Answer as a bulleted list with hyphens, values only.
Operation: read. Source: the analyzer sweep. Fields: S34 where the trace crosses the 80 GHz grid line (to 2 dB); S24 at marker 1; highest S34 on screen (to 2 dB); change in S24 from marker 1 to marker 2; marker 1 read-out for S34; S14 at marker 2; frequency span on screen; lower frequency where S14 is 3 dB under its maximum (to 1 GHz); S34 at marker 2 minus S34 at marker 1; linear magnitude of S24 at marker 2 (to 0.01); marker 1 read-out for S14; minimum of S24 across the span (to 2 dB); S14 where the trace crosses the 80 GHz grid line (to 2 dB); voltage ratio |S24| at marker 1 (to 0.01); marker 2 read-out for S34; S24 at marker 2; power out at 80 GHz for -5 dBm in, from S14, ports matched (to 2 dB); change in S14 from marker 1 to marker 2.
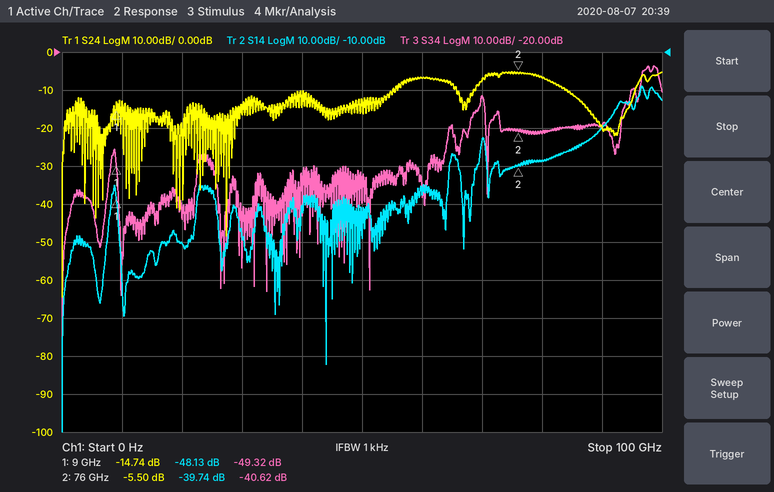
- -42 dB
- -14.74 dB
- -24 dB
- 9.24 dB
- -49.32 dB
- -39.74 dB
- 100 GHz
- 96 GHz
- 8.70 dB
- 0.53
- -48.13 dB
- -64 dB
- -38 dB
- 0.18
- -40.62 dB
- -5.50 dB
- -44 dBm
- 8.39 dB
